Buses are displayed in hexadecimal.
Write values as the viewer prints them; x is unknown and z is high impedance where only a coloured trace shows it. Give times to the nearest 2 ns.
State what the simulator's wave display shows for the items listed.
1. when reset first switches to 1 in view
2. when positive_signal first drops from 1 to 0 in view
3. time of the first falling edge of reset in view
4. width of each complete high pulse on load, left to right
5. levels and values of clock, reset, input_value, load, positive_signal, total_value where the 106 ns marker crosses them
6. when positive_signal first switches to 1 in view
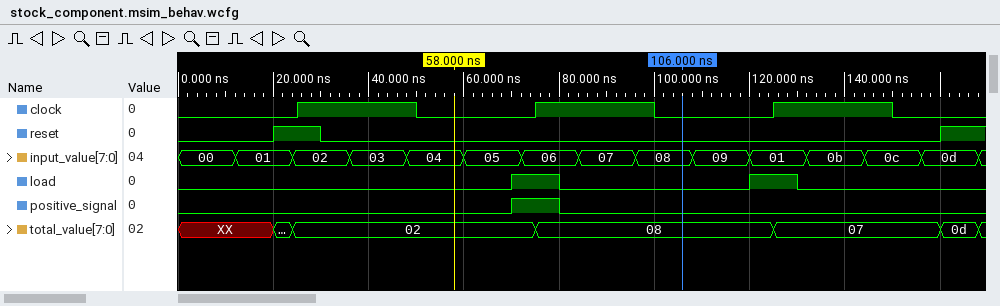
20 ns
80 ns
30 ns
10 ns, 10 ns
clock=0, reset=0, input_value=08, load=0, positive_signal=0, total_value=08
70 ns
